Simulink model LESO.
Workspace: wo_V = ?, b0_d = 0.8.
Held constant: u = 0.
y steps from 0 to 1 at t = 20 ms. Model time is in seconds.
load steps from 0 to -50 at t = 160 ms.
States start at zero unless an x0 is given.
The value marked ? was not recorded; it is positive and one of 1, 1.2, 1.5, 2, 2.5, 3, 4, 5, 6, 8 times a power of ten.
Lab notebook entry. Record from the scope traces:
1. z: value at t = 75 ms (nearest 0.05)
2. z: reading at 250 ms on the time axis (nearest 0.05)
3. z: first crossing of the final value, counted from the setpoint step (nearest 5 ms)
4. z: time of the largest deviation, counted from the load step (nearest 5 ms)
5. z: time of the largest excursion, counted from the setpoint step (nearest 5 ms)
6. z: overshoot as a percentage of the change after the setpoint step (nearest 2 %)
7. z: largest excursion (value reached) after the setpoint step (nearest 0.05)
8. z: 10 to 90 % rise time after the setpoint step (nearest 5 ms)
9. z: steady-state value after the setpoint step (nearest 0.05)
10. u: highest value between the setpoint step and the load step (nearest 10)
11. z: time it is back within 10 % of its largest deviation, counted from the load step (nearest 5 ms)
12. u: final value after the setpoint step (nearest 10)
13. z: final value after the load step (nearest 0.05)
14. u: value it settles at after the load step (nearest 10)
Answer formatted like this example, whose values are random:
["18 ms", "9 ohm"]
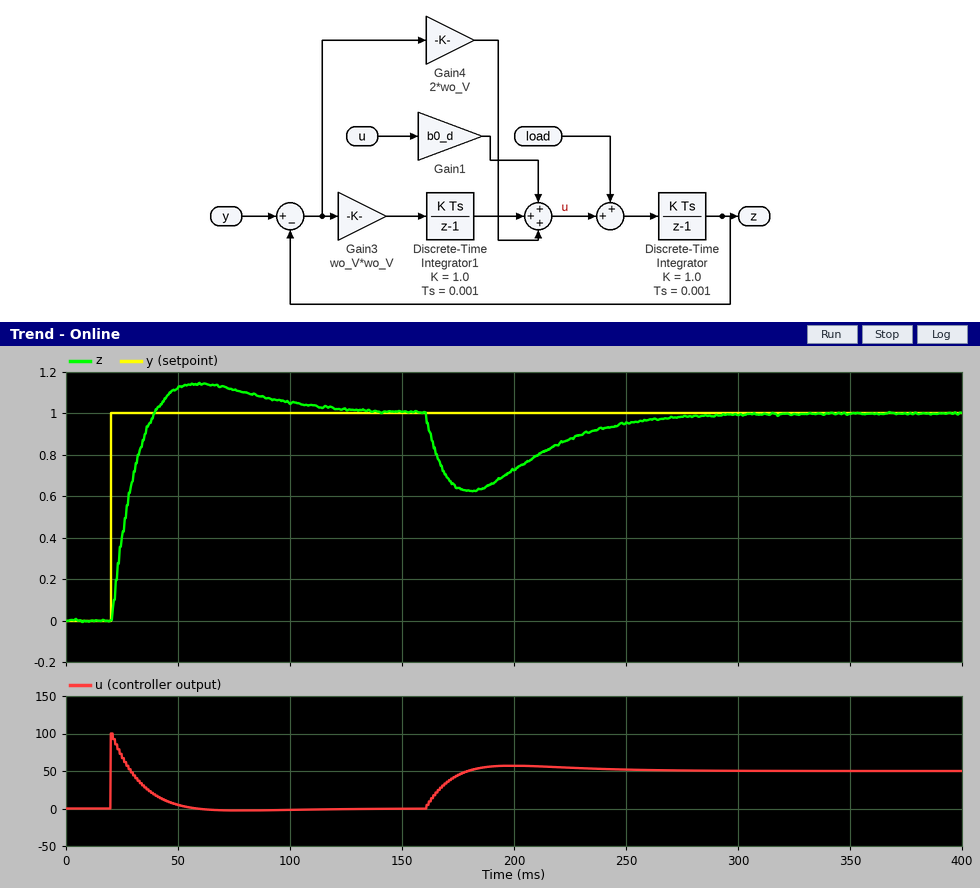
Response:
["1.10", "0.95", "20 ms", "20 ms", "40 ms", "14 %", "1.15", "15 ms", "1.00", "100", "95 ms", "0", "1.00", "50"]
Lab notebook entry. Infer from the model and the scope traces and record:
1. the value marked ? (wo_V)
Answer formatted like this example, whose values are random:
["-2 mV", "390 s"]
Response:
["50"]
